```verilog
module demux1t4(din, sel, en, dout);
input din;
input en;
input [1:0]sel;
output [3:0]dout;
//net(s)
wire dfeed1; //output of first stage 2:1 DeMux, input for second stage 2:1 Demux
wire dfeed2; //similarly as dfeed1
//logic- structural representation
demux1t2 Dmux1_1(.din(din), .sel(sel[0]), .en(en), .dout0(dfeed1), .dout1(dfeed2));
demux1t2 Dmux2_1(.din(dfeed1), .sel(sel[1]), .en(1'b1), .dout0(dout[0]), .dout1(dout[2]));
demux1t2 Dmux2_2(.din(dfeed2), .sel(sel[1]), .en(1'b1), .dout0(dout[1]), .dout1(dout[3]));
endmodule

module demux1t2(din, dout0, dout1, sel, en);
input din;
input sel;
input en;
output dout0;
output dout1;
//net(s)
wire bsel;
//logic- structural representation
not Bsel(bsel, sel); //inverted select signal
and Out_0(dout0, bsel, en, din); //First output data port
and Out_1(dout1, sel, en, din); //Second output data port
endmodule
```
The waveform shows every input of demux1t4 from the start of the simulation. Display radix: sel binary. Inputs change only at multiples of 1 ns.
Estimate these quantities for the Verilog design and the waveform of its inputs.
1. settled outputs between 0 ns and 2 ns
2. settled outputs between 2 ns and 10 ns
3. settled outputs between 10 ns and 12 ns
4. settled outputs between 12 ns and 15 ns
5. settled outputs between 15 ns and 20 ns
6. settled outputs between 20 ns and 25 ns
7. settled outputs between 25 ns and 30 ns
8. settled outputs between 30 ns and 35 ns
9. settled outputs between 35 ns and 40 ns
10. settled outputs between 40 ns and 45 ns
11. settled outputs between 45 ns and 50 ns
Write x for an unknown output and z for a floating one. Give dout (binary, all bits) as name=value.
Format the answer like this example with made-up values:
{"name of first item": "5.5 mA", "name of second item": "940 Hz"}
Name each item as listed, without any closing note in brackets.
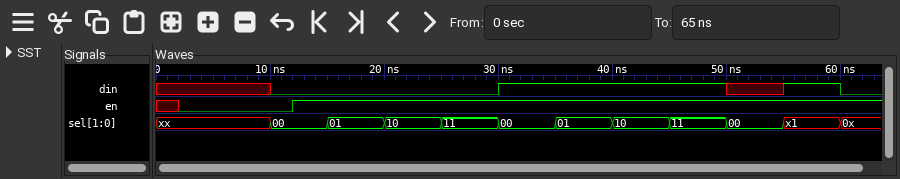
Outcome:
{"settled outputs between 0 ns and 2 ns": "dout=x", "settled outputs between 2 ns and 10 ns": "dout=0000", "settled outputs between 10 ns and 12 ns": "dout=0000", "settled outputs between 12 ns and 15 ns": "dout=0000", "settled outputs between 15 ns and 20 ns": "dout=0000", "settled outputs between 20 ns and 25 ns": "dout=0000", "settled outputs between 25 ns and 30 ns": "dout=0000", "settled outputs between 30 ns and 35 ns": "dout=0001", "settled outputs between 35 ns and 40 ns": "dout=0010", "settled outputs between 40 ns and 45 ns": "dout=0100", "settled outputs between 45 ns and 50 ns": "dout=1000"}
